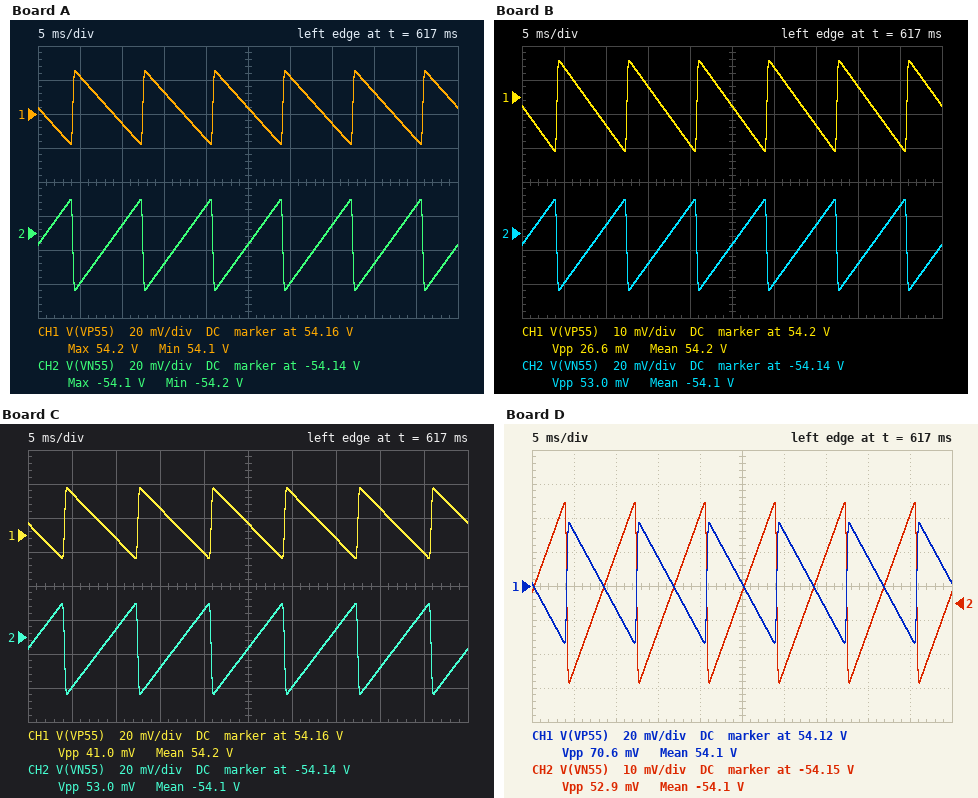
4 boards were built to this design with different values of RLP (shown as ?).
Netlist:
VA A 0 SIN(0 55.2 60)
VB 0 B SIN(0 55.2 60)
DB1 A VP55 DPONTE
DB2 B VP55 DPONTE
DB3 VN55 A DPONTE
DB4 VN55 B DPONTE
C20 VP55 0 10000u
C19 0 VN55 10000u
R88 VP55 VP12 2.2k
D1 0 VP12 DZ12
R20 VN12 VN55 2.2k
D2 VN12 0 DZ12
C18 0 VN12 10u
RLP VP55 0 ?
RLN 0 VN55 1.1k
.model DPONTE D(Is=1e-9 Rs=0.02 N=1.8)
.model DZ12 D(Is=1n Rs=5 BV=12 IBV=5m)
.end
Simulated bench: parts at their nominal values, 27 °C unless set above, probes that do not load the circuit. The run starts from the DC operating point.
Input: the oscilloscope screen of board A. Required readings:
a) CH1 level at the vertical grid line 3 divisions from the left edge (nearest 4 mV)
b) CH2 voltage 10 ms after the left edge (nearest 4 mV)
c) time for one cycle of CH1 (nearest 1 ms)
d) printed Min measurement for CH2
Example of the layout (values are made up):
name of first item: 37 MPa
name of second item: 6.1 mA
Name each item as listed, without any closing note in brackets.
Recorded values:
CH1 level at the vertical grid line 3 divisions from the left edge: 54.172 V
CH2 voltage 10 ms after the left edge: -54.136 V
time for one cycle of CH1: 8 ms
printed Min measurement for CH2: -54.2 V
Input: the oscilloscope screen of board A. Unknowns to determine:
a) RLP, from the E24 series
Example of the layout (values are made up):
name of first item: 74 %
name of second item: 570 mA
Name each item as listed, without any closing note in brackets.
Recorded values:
RLP, from the E24 series: 1.5 kΩ
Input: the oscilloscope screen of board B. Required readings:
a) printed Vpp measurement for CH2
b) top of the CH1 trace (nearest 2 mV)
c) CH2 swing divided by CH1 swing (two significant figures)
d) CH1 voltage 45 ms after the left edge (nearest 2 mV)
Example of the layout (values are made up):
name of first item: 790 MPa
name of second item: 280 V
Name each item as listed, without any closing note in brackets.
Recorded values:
printed Vpp measurement for CH2: 53.0 mV
top of the CH1 trace: 54.210 V
CH2 swing divided by CH1 swing: 2.0
CH1 voltage 45 ms after the left edge: 54.186 V
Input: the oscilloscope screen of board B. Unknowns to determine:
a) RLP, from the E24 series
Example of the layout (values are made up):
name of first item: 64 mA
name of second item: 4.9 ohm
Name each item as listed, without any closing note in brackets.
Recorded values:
RLP, from the E24 series: 3.6 kΩ
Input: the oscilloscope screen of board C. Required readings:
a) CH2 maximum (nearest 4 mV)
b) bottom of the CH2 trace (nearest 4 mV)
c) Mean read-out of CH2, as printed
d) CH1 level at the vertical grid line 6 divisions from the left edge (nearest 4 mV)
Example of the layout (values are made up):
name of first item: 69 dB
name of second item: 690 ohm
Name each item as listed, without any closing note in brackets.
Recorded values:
CH2 maximum: -54.120 V
bottom of the CH2 trace: -54.172 V
Mean read-out of CH2, as printed: -54.1 V
CH1 level at the vertical grid line 6 divisions from the left edge: 54.184 V
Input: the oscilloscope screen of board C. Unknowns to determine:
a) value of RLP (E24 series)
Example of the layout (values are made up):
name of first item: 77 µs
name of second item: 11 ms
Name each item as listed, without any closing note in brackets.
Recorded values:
value of RLP: 1.6 kΩ
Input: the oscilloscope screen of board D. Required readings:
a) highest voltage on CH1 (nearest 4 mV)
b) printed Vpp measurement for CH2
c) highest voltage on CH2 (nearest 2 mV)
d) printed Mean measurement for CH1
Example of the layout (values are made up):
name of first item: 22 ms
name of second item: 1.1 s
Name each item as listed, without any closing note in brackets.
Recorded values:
highest voltage on CH1: 54.156 V
printed Vpp measurement for CH2: 52.9 mV
highest voltage on CH2: -54.120 V
printed Mean measurement for CH1: 54.1 V
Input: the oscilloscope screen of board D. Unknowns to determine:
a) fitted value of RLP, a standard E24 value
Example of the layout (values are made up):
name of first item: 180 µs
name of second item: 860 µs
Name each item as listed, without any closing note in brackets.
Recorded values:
fitted value of RLP, a standard E24 value: 750 Ω
